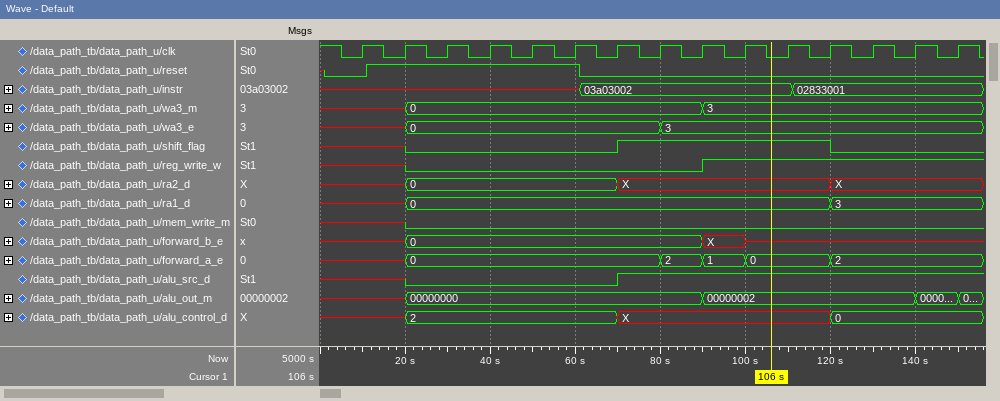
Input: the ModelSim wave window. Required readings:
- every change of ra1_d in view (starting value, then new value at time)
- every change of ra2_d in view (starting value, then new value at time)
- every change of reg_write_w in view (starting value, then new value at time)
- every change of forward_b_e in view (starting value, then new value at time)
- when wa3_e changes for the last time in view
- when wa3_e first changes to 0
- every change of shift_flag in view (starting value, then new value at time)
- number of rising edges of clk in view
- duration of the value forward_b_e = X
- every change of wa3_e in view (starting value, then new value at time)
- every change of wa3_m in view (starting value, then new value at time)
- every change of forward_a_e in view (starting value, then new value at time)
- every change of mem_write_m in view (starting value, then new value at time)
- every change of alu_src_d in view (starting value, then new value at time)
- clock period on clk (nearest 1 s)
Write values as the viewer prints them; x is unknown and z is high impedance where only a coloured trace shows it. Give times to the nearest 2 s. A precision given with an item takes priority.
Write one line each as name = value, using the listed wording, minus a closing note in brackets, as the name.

every change of ra1_d in view = x, 0 at 20 s, 3 at 120 s
every change of ra2_d in view = x, 0 at 20 s, X at 70 s, X at 120 s
every change of reg_write_w in view = x, 0 at 20 s, 1 at 90 s
every change of forward_b_e in view = x, 0 at 20 s, X at 90 s, x at 100 s
when wa3_e changes for the last time in view = 80 s
when wa3_e first changes to 0 = 20 s
every change of shift_flag in view = x, 0 at 20 s, 1 at 70 s, 0 at 120 s
number of rising edges of clk in view = 15
duration of the value forward_b_e = X = 10 s
every change of wa3_e in view = x, 0 at 20 s, 3 at 80 s
every change of wa3_m in view = x, 0 at 20 s, 3 at 90 s
every change of forward_a_e in view = x, 0 at 20 s, 2 at 80 s, 1 at 90 s, 0 at 100 s, 2 at 120 s
every change of mem_write_m in view = x, 0 at 20 s
every change of alu_src_d in view = x, 0 at 20 s, 1 at 70 s
clock period on clk = 10 s
